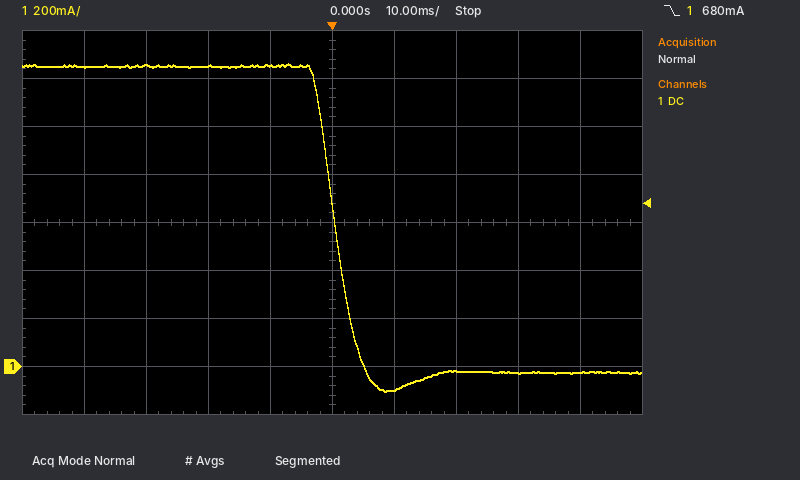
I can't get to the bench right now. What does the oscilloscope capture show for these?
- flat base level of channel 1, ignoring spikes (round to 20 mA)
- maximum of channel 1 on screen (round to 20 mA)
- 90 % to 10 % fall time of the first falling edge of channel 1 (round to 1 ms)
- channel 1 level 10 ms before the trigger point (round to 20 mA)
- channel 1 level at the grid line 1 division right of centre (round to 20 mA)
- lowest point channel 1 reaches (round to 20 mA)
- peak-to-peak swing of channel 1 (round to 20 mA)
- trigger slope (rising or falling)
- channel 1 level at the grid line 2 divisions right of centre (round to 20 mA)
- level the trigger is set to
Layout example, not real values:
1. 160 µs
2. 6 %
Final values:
1. -20 mA
2. 1.26 A
3. 6 ms
4. 1.26 A
5. -100 mA
6. -100 mA
7. 1.36 A
8. falling
9. -20 mA
10. 680 mA
